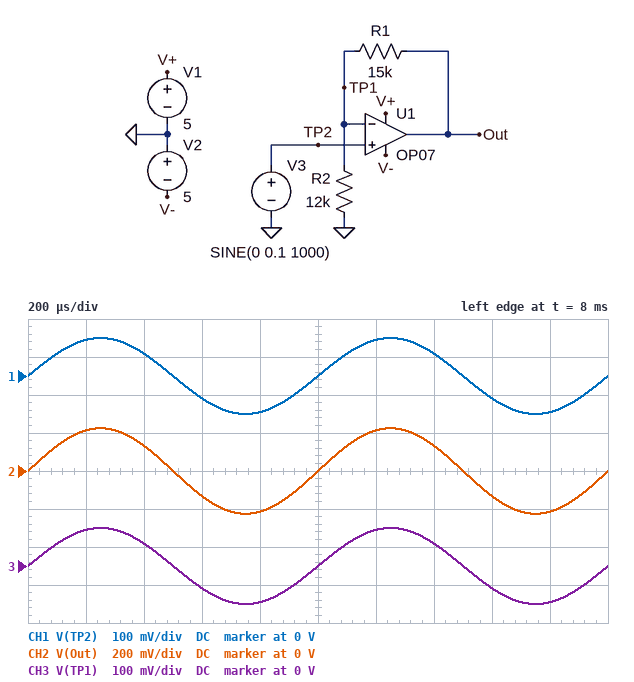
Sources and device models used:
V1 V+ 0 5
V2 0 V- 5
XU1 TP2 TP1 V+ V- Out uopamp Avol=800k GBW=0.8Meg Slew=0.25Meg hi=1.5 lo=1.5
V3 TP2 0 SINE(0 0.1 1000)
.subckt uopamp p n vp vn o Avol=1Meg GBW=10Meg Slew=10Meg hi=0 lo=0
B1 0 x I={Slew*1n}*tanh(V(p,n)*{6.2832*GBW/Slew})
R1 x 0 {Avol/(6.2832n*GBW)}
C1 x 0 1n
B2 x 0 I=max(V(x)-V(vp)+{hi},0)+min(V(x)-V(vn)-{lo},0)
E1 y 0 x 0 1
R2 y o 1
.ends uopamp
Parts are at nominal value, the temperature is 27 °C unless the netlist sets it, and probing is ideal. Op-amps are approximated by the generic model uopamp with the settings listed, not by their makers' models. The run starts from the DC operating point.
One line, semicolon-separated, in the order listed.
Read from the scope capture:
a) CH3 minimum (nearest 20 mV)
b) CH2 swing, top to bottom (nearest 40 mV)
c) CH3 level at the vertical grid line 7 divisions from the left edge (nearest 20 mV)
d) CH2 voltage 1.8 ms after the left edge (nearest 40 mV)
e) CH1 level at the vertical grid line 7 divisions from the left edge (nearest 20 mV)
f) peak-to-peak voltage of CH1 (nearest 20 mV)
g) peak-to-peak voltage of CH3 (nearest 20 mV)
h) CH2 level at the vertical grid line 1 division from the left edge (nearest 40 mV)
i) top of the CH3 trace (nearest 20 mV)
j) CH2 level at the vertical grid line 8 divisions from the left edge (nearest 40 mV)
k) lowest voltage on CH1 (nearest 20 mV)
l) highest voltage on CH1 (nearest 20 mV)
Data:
-100 mV; 440 mV; 60 mV; -200 mV; 60 mV; 200 mV; 200 mV; 200 mV; 100 mV; -120 mV; -100 mV; 100 mV
